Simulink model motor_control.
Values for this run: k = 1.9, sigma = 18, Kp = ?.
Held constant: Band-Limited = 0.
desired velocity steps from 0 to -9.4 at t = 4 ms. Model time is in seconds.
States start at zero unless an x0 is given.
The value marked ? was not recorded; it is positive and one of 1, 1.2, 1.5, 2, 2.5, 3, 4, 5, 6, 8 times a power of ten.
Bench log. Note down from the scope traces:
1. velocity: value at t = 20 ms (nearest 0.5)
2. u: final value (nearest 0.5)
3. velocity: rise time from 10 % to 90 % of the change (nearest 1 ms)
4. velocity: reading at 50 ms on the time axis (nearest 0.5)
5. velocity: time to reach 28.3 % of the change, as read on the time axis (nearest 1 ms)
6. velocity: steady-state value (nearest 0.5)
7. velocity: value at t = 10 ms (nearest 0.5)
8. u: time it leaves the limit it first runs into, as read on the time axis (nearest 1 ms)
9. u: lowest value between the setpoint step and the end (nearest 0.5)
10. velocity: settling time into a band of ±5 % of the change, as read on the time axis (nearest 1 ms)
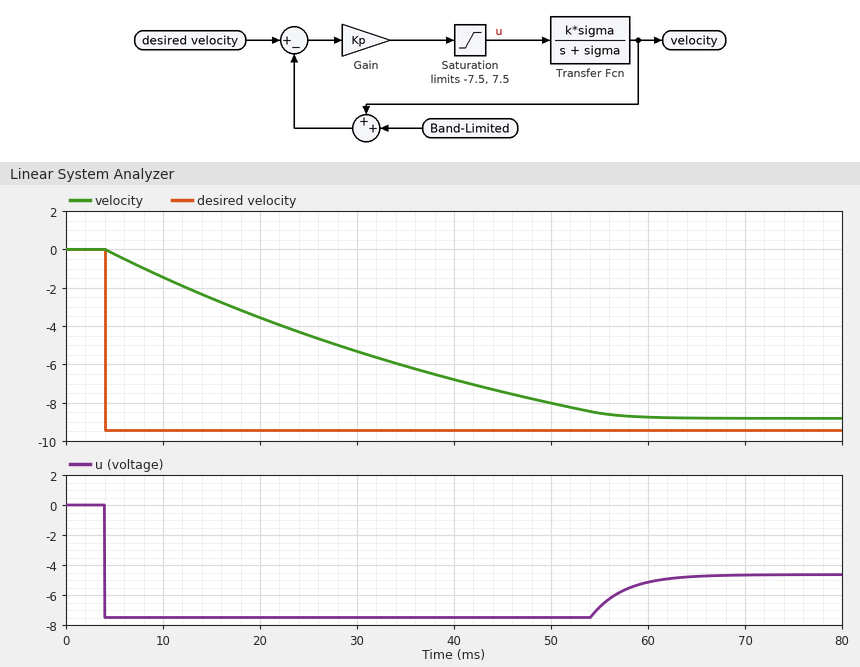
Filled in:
-3.5
-4.5
42 ms
-8.0
15 ms
-9.0
-1.5
54 ms
-7.5
53 ms
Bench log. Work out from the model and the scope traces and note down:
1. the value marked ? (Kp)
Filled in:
8
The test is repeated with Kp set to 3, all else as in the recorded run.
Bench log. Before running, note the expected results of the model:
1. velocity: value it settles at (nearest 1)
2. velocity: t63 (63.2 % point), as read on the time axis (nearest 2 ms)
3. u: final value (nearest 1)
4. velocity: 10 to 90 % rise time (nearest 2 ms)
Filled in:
-8
28 ms
-4
36 ms
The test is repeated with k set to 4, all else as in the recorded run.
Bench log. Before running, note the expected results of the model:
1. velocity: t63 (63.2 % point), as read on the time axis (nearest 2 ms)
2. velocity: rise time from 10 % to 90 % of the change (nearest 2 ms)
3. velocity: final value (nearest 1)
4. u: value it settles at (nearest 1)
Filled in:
16 ms
16 ms
-9
-2
